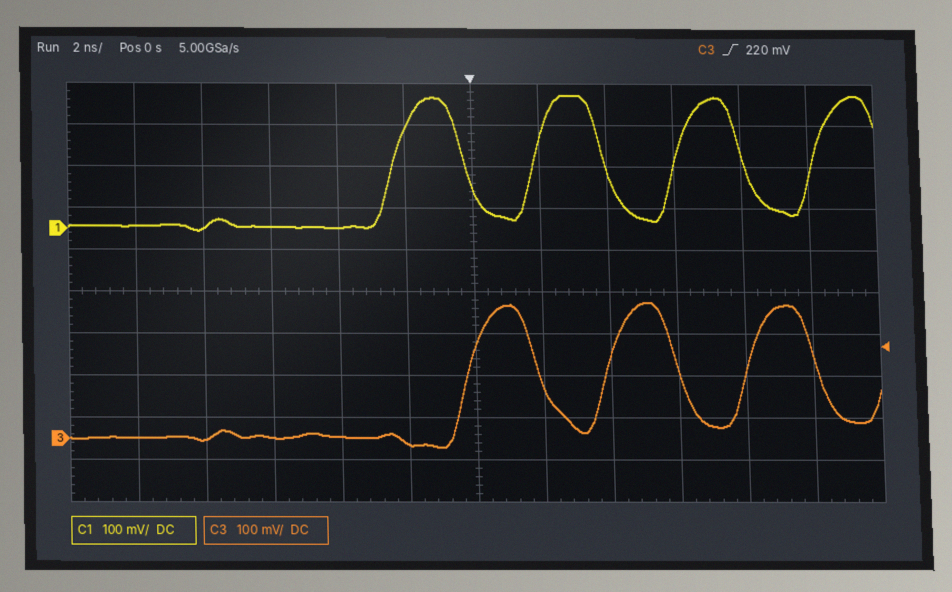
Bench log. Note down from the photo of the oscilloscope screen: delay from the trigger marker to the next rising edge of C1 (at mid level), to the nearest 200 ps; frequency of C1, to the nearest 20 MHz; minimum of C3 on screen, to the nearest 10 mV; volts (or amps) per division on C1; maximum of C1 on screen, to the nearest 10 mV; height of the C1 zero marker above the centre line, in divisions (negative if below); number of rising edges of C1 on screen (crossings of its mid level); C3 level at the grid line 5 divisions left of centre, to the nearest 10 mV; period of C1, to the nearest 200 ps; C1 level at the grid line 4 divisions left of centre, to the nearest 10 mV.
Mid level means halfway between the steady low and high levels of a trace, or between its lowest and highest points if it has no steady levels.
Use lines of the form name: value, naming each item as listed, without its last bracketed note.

delay from the trigger marker to the next rising edge of C1 (at mid level), to the nearest 200 ps: 1.8 ns
frequency of C1, to the nearest 20 MHz: 240 MHz
minimum of C3 on screen, to the nearest 10 mV: -20 mV
volts (or amps) per division on C1: 100 mV
maximum of C1 on screen, to the nearest 10 mV: 320 mV
height of the C1 zero marker above the centre line, in divisions: +1.5 div
number of rising edges of C1 on screen: 4
C3 level at the grid line 5 divisions left of centre, to the nearest 10 mV: 0 mV
period of C1, to the nearest 200 ps: 4.2 ns
C1 level at the grid line 4 divisions left of centre, to the nearest 10 mV: 0 mV
